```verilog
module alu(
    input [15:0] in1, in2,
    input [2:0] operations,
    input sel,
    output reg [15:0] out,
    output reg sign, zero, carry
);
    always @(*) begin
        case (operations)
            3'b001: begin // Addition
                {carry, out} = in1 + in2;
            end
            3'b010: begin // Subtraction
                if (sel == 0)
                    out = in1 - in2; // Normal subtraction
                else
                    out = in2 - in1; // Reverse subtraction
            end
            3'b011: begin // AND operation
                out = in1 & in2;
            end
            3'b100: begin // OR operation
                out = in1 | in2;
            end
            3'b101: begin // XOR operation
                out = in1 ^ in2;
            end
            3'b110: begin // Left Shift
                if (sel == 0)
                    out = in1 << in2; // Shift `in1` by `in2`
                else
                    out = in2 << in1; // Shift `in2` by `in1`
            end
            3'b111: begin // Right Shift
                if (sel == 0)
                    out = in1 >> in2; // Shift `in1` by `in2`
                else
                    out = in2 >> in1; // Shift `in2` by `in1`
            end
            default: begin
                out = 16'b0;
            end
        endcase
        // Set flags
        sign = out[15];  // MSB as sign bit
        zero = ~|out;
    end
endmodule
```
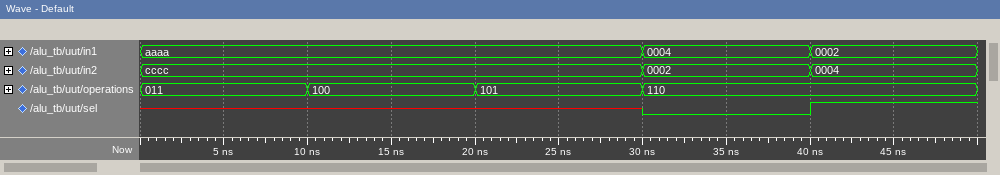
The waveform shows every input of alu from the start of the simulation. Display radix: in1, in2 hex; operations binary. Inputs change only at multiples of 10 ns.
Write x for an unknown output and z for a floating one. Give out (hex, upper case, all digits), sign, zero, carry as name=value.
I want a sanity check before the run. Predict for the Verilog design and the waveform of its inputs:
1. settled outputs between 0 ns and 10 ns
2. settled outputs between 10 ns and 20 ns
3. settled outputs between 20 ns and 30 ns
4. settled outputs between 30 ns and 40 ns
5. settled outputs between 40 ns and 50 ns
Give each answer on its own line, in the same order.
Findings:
out=8888, sign=1, zero=0, carry=x
out=EEEE, sign=1, zero=0, carry=x
out=6666, sign=0, zero=0, carry=x
out=0010, sign=0, zero=0, carry=x
out=0010, sign=0, zero=0, carry=x
